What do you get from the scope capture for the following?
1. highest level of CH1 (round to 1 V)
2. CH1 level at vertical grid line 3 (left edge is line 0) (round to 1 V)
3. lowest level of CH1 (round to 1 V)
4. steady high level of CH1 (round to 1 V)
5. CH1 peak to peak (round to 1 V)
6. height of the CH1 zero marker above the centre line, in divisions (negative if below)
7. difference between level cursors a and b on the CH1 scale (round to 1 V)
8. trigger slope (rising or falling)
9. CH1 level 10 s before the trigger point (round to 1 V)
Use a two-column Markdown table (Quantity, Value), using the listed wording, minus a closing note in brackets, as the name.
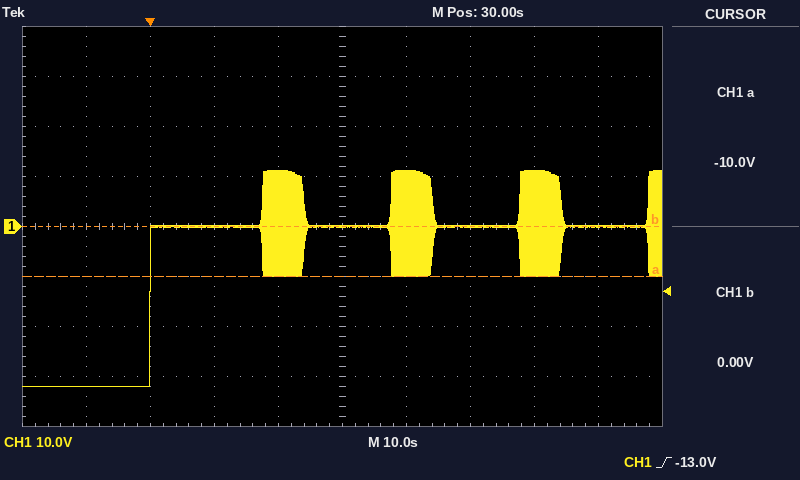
| Quantity | Value |
|---|---|
| highest level of CH1 | 11 V |
| CH1 level at vertical grid line 3 (left edge is line 0) | 0 V |
| lowest level of CH1 | -32 V |
| steady high level of CH1 | 0 V |
| CH1 peak to peak | 43 V |
| height of the CH1 zero marker above the centre line, in divisions | 0.0 div |
| difference between level cursors a and b on the CH1 scale | 10 V |
| trigger slope | rising |
| CH1 level 10 s before the trigger point | -32 V |
